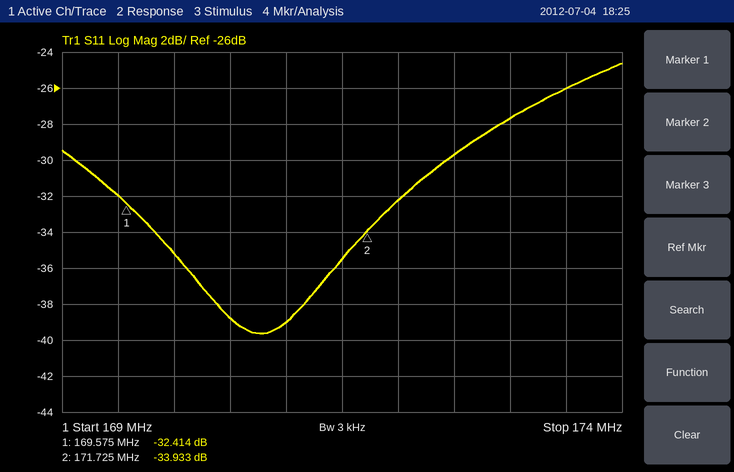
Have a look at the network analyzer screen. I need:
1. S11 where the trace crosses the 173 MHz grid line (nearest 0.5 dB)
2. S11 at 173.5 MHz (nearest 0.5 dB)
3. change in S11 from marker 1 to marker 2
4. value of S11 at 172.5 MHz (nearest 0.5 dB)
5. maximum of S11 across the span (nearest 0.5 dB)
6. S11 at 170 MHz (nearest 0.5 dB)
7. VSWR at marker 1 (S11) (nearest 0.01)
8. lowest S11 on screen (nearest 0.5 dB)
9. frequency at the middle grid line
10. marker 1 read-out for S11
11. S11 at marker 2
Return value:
-27.5 dB
-26.0 dB
-1.519 dB
-29.5 dB
-24.5 dB
-35.0 dB
1.05
-39.5 dB
171.5 MHz
-32.414 dB
-33.933 dB
